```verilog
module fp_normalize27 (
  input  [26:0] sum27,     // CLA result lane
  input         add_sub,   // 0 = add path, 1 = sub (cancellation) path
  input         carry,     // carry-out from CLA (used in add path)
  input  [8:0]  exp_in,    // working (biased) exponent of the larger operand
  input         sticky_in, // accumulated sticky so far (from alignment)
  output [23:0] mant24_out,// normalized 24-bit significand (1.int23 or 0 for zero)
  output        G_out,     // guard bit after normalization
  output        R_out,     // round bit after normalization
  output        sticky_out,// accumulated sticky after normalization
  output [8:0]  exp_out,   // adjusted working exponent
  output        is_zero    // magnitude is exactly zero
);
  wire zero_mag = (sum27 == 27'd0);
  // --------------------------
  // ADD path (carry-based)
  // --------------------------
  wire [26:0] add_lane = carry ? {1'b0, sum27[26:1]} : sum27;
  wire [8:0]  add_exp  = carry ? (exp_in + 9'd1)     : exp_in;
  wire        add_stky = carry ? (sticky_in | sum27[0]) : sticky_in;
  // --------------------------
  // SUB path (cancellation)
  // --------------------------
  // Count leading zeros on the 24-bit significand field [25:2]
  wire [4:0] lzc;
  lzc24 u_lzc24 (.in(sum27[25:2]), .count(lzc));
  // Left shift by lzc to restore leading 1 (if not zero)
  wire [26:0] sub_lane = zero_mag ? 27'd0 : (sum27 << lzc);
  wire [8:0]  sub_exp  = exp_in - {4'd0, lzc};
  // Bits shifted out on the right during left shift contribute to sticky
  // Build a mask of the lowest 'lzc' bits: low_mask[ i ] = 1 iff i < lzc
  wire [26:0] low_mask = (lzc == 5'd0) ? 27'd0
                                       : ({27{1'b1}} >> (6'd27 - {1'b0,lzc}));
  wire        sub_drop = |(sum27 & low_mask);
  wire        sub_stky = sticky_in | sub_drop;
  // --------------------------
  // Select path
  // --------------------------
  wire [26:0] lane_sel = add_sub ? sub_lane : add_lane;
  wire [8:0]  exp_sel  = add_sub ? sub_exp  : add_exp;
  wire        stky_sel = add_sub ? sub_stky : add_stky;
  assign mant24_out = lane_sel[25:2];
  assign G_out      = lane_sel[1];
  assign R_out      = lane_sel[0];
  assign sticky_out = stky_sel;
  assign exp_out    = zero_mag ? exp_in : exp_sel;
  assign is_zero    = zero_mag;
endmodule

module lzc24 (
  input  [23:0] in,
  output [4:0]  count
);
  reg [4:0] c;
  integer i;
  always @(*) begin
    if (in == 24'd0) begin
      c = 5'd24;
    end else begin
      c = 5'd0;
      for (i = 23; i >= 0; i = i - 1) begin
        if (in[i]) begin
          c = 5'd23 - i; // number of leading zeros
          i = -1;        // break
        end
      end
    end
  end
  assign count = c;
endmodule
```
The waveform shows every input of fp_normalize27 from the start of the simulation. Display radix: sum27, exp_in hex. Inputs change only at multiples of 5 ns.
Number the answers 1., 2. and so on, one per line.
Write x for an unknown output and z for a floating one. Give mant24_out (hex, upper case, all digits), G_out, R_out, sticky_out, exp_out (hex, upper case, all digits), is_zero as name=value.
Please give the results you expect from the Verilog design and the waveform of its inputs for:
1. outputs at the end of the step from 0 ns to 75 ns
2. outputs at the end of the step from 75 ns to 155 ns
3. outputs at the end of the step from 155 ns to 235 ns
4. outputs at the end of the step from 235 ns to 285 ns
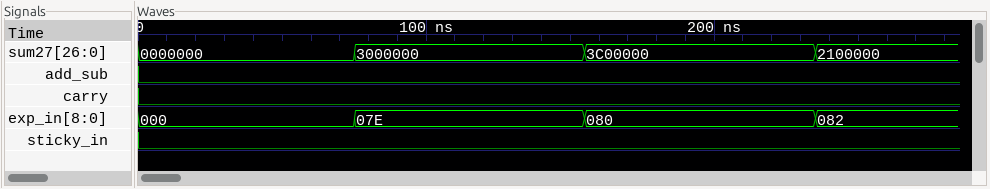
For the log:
1. mant24_out=000000, G_out=0, R_out=0, sticky_out=0, exp_out=000, is_zero=1
2. mant24_out=C00000, G_out=0, R_out=0, sticky_out=0, exp_out=07E, is_zero=0
3. mant24_out=F00000, G_out=0, R_out=0, sticky_out=0, exp_out=080, is_zero=0
4. mant24_out=840000, G_out=0, R_out=0, sticky_out=0, exp_out=082, is_zero=0
